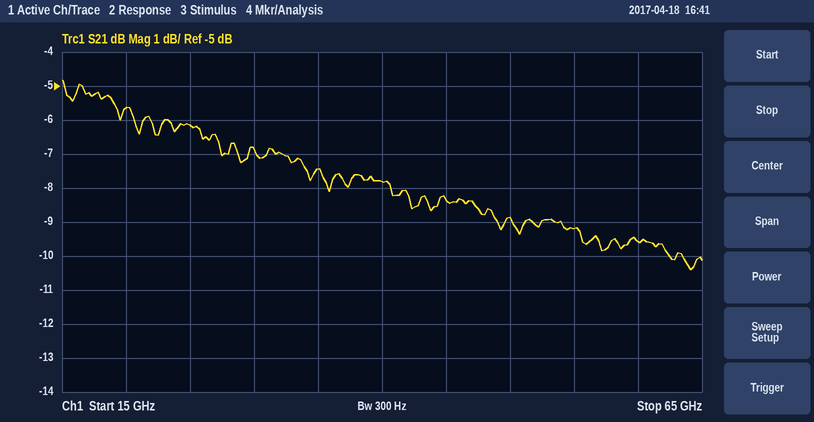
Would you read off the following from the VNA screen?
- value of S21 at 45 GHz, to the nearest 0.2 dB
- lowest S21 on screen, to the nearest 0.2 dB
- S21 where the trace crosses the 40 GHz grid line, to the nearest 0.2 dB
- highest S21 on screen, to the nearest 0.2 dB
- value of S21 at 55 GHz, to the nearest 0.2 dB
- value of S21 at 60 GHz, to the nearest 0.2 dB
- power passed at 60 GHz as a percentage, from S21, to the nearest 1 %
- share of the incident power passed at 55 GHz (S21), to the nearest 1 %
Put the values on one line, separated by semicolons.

-8.4 dB; -10.4 dB; -7.8 dB; -4.8 dB; -9.2 dB; -9.6 dB; 11 %; 12 %
